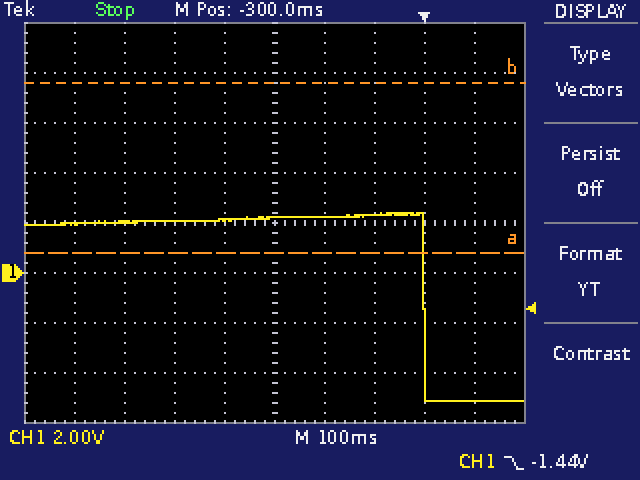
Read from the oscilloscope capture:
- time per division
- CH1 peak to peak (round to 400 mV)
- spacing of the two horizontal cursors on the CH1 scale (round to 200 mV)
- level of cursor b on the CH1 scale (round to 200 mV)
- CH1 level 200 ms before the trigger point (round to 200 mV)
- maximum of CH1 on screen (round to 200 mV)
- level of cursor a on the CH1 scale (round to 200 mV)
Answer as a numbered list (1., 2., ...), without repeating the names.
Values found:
1. 100 ms
2. 7.6 V
3. 6.8 V
4. 7.6 V
5. 2.2 V
6. 2.4 V
7. 800 mV
